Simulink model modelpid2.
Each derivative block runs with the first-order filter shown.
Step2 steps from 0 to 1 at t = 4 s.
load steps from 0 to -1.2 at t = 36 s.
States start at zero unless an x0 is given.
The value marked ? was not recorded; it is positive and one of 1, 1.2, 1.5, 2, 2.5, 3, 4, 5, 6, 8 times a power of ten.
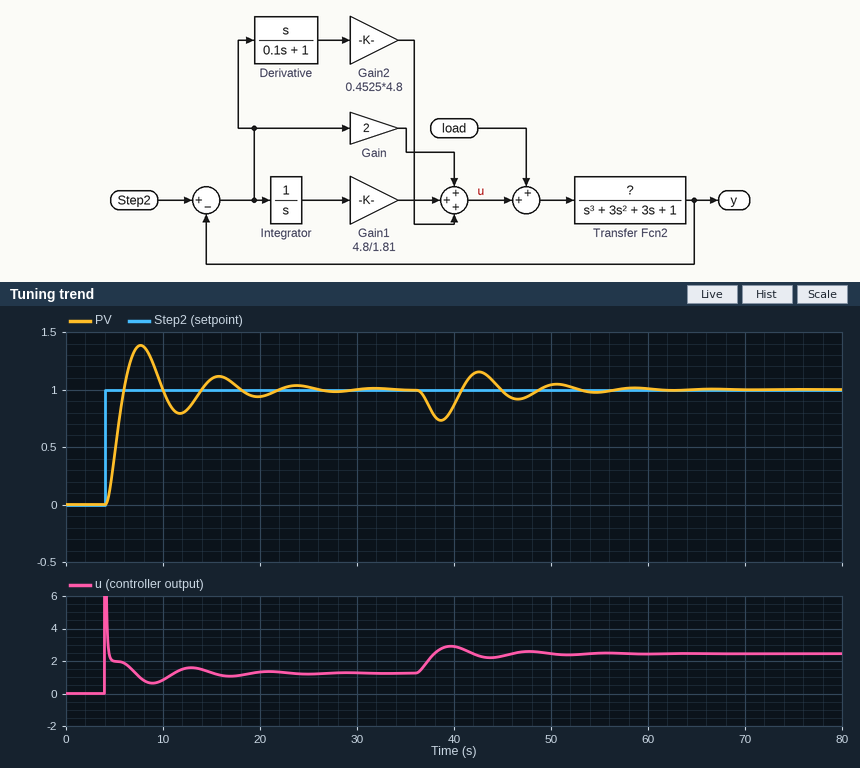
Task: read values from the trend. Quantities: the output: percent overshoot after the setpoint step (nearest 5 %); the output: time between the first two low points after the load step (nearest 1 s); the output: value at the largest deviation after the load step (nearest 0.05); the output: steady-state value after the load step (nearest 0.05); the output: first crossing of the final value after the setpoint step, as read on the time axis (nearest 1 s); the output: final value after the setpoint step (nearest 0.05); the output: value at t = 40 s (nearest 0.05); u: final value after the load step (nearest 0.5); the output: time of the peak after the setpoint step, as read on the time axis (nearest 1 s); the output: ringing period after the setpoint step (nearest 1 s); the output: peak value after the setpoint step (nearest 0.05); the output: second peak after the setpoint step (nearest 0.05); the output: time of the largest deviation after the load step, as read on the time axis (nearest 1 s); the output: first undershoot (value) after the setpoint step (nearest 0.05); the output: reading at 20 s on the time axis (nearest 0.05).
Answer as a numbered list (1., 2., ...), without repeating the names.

1. 40 %
2. 8 s
3. 0.75
4. 1.00
5. 6 s
6. 1.00
7. 0.85
8. 2.5
9. 8 s
10. 8 s
11. 1.40
12. 1.10
13. 39 s
14. 0.80
15. 0.95
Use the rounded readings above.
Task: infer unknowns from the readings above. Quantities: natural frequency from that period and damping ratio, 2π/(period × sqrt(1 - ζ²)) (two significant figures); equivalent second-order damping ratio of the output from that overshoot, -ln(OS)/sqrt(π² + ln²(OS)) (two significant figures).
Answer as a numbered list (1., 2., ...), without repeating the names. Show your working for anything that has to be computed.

1. 2π / (8 × sqrt(1 - 0.28²)) = 0.82 rad/s
2. ln(0.4) = -0.916; 0.916 / sqrt(9.870 + 0.840) = 0.28
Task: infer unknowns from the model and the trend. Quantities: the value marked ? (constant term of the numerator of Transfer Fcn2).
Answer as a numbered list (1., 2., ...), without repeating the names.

1. 0.8
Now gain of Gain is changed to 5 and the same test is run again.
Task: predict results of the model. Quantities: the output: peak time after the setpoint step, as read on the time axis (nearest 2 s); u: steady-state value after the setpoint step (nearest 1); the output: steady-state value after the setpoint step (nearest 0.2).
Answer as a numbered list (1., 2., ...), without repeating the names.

1. 6 s
2. 1
3. 1.0
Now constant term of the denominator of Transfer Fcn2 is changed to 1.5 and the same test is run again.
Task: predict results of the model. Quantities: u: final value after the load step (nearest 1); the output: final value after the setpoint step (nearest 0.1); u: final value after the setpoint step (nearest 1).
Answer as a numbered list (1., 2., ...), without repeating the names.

1. 3
2. 1.0
3. 2
